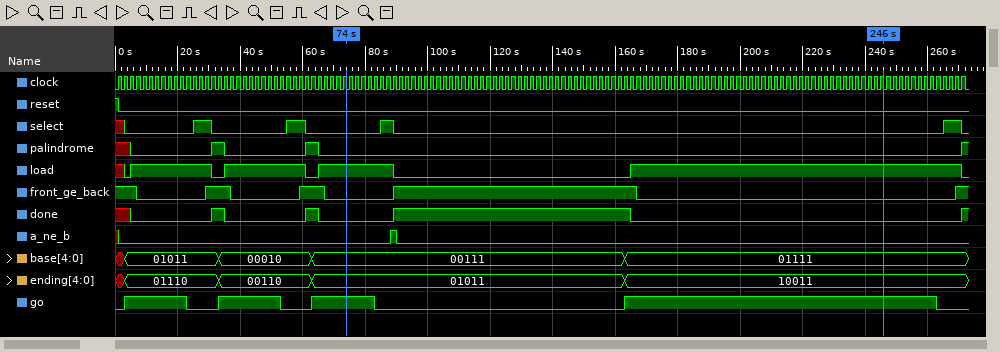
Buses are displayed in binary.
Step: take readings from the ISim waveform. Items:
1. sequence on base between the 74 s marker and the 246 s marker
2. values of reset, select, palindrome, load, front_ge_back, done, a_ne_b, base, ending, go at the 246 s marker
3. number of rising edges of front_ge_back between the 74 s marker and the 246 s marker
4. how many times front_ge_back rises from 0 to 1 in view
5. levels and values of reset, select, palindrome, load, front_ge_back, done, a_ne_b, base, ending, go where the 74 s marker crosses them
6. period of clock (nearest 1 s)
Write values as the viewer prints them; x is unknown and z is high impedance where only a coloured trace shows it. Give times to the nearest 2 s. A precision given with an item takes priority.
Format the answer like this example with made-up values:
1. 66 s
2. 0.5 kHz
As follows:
1. 00111, 01111
2. reset=0, select=0, palindrome=0, load=1, front_ge_back=0, done=0, a_ne_b=0, base=01111, ending=10011, go=1
3. 1
4. 4
5. reset=0, select=0, palindrome=0, load=1, front_ge_back=0, done=0, a_ne_b=0, base=00111, ending=01011, go=1
6. 2 s
